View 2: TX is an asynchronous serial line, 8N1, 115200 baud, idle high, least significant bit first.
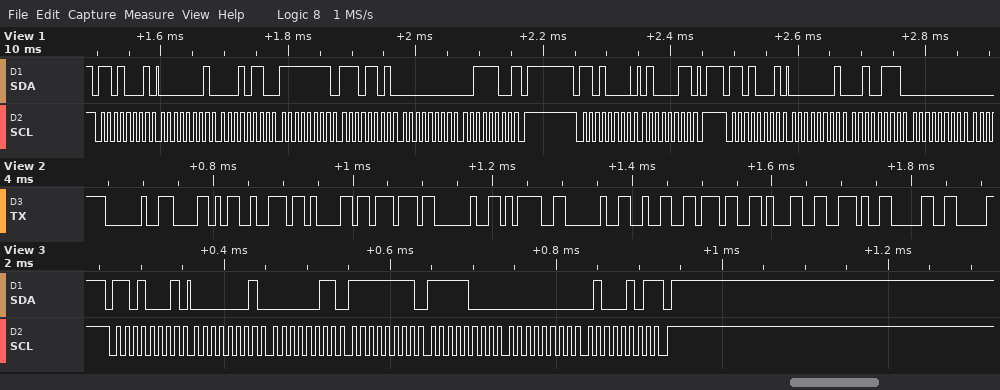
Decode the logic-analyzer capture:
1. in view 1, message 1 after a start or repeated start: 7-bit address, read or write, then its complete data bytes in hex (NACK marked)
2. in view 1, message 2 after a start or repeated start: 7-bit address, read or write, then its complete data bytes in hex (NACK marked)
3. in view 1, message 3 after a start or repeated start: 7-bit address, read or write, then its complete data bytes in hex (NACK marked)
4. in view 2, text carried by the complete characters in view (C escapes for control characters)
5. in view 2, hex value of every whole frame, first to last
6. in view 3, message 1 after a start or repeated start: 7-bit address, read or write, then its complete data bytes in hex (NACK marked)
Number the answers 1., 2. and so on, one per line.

1. 0x68 read: 01 16 FF ED 00 3C NACK
2. 0x68 write: 43
3. 0x68 read: 01 27 00
4. " Xraw = 271.0"
5. 20 58 72 61 77 20 3D 20 32 37 31 2E 30
6. 0x68 read: 01 03 FF F8 00 45 NACK
